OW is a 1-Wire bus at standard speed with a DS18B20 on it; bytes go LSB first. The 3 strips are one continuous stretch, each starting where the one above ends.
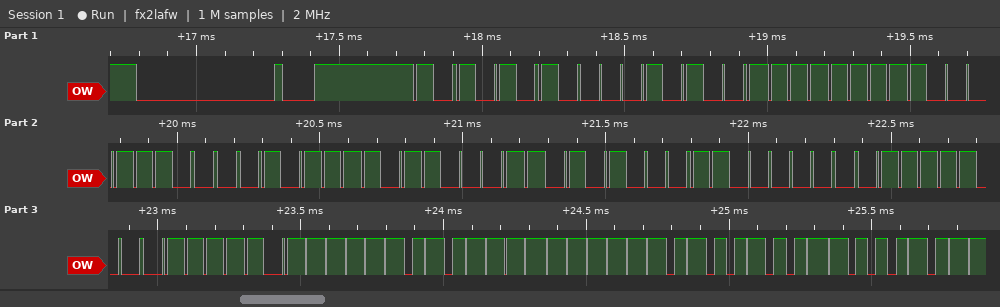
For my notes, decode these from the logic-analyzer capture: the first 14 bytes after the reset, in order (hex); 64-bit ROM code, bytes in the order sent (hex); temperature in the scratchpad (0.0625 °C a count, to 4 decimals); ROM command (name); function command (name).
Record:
55 28 FF 71 E8 8D 15 03 3E BE 5F FF 4B 46
28 FF 71 E8 8D 15 03 3E
-10.0625 °C
Match ROM
Read Scratchpad
